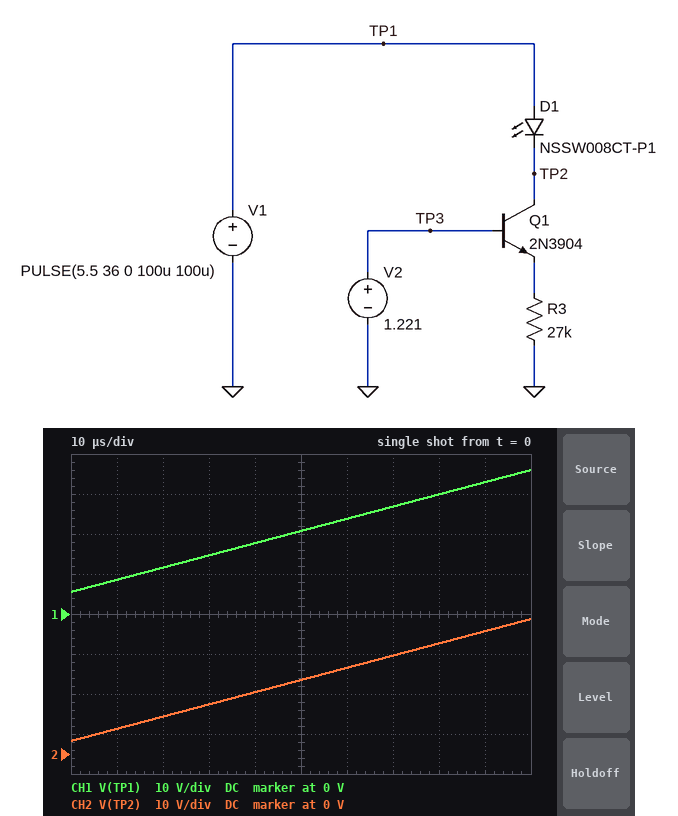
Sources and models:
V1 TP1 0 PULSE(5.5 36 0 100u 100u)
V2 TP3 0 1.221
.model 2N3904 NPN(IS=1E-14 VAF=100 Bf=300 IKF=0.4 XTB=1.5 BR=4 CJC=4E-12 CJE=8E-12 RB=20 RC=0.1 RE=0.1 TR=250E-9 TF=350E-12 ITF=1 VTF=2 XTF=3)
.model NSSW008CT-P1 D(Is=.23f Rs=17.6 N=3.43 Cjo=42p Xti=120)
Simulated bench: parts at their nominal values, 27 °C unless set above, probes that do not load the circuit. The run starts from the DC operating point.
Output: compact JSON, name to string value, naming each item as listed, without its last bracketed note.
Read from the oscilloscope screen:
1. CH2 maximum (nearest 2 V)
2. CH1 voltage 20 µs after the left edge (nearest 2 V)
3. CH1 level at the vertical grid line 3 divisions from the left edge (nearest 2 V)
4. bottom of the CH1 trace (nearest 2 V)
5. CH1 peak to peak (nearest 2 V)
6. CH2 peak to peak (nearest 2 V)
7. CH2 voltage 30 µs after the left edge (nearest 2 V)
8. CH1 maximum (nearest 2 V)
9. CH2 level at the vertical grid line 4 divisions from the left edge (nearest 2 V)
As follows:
{"CH2 maximum": "34 V", "CH1 voltage 20 µs after the left edge": "12 V", "CH1 level at the vertical grid line 3 divisions from the left edge": "14 V", "bottom of the CH1 trace": "6 V", "CH1 peak to peak": "30 V", "CH2 peak to peak": "30 V", "CH2 voltage 30 µs after the left edge": "12 V", "CH1 maximum": "36 V", "CH2 level at the vertical grid line 4 divisions from the left edge": "16 V"}
